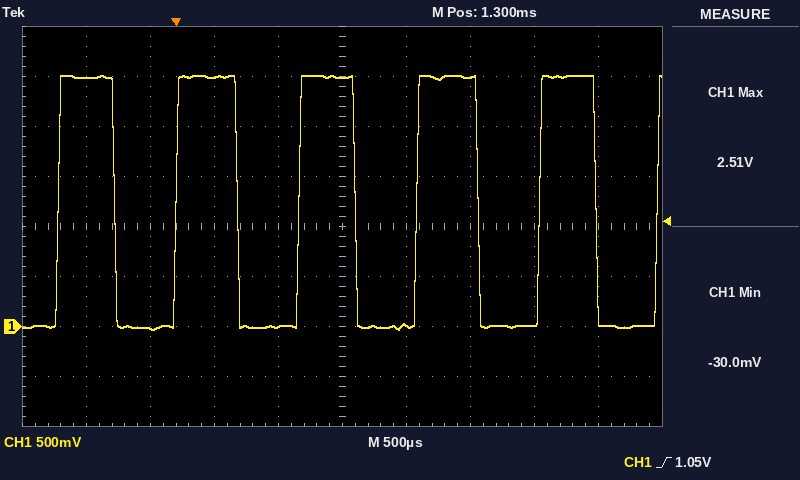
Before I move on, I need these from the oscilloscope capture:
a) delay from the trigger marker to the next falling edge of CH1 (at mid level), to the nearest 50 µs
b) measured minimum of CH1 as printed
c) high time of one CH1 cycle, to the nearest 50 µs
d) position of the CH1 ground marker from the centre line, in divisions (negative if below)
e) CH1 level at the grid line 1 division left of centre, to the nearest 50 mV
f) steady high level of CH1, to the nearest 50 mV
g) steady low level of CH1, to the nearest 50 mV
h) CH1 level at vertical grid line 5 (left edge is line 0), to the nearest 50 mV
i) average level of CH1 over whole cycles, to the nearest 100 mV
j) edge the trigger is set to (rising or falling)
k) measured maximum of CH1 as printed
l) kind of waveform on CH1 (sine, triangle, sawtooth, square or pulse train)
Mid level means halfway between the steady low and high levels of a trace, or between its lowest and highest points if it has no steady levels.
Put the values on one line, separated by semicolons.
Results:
500 µs; -30.0 mV; 450 µs; -2.0 div; 0 mV; 2.50 V; 0 mV; 2.50 V; 1.2 V; rising; 2.51 V; square
